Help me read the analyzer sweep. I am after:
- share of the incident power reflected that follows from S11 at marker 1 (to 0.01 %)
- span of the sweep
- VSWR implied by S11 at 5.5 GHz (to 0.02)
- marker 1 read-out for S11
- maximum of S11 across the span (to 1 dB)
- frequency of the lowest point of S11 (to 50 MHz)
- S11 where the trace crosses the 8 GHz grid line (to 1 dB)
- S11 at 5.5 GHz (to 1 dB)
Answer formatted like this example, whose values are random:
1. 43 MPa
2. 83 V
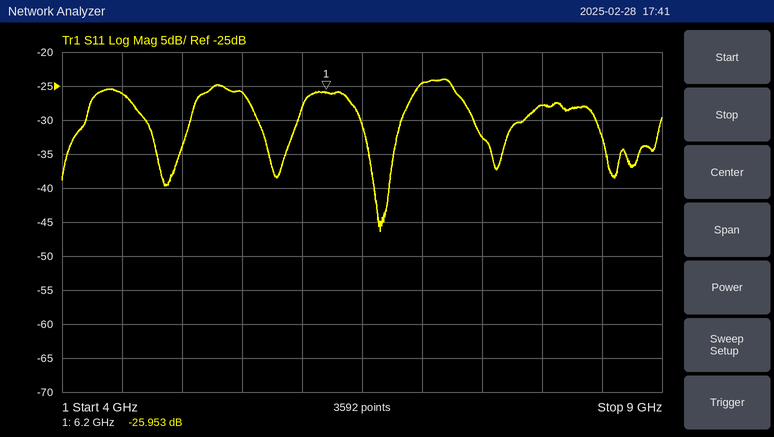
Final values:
1. 0.25 %
2. 5 GHz
3. 1.10
4. -25.953 dB
5. -24 dB
6. 6.65 GHz
7. -28 dB
8. -26 dB
